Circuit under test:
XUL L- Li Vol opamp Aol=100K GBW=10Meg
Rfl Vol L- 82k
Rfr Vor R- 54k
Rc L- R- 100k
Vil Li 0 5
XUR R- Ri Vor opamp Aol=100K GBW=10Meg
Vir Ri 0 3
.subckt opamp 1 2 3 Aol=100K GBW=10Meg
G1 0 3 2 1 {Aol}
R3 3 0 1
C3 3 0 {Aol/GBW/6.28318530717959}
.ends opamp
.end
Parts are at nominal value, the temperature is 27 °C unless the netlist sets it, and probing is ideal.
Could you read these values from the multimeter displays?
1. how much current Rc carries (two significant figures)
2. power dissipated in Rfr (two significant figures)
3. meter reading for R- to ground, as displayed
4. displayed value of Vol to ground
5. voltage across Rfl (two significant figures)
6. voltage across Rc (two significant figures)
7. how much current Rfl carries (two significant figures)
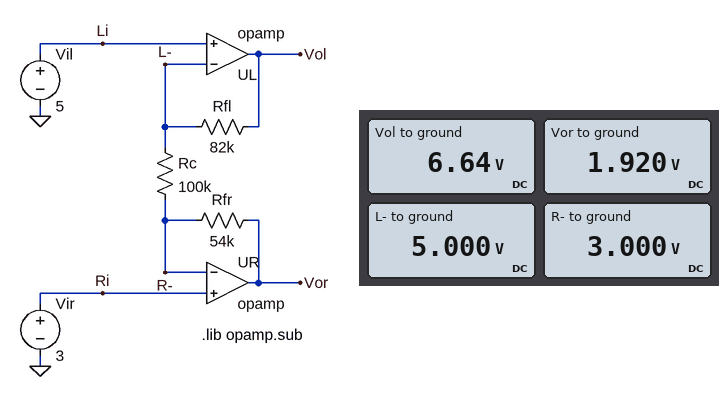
20 µA
22 µW
3.000 V
6.64 V
1.6 V
2.0 V
20 µA
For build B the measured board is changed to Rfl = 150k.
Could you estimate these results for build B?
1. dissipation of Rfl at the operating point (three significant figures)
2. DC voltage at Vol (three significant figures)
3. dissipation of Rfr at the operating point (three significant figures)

60.0 µW
8.00 V
21.6 µW
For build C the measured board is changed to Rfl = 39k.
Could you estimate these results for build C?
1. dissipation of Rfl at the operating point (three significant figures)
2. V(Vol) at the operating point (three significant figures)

15.6 µW
5.78 V
